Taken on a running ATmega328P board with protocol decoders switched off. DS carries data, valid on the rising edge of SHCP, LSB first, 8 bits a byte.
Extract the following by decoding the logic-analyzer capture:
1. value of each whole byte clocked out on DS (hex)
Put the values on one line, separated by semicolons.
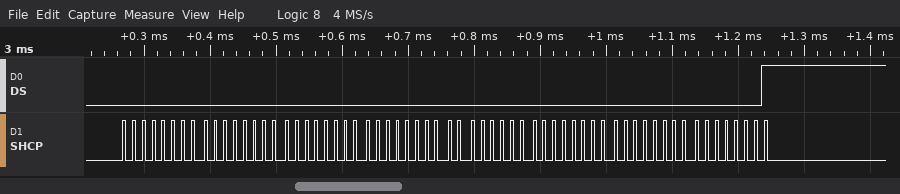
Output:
00 00 00 00 00 00 00 80
